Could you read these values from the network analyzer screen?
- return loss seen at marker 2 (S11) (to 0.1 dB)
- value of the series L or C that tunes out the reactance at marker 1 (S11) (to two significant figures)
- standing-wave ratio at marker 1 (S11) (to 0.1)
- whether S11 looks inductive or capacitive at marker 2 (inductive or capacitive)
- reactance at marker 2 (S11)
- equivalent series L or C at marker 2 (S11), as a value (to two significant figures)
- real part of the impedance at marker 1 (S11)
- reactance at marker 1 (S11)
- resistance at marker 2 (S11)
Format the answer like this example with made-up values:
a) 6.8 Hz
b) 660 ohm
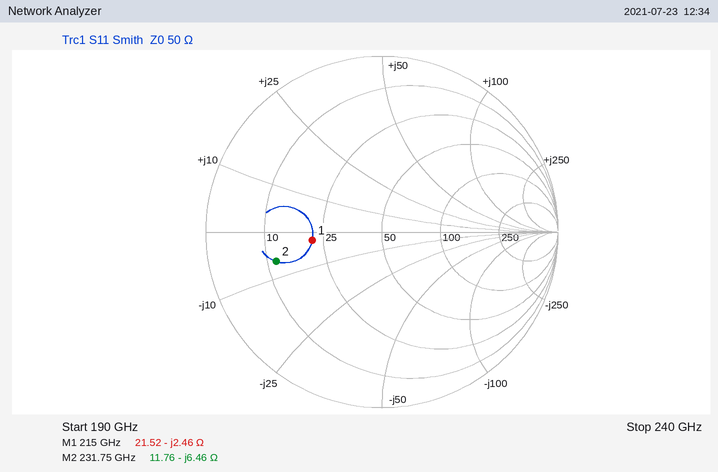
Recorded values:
a) 4.1 dB
b) 1.8 pH
c) 2.3
d) capacitive
e) -6.46 Ω
f) 110 fF
g) 21.52 Ω
h) -2.46 Ω
i) 11.76 Ω
